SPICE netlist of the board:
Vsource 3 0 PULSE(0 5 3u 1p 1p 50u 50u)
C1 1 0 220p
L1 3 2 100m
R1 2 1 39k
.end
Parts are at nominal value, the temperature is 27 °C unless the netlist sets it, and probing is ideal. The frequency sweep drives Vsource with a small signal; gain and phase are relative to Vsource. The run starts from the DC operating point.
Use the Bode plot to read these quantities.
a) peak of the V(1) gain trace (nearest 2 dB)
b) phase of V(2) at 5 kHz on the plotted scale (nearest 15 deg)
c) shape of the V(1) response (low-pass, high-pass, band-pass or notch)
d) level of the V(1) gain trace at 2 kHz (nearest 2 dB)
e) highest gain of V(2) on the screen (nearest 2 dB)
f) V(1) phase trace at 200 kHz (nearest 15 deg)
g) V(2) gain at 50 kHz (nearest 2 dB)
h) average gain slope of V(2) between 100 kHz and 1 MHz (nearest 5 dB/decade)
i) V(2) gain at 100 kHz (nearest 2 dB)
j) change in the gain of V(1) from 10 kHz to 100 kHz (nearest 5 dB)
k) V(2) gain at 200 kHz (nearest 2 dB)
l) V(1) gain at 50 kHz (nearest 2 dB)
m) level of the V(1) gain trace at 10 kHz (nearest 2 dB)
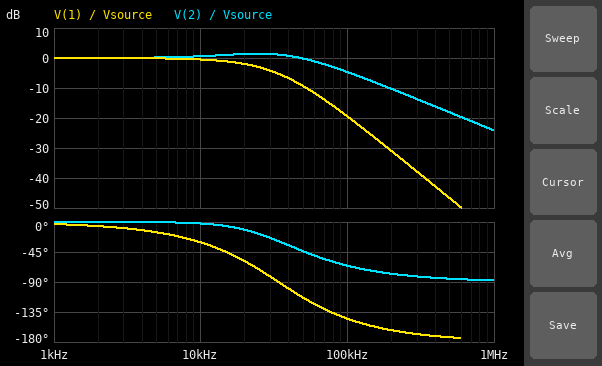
0 dB
0 deg
low-pass
0 dB
2 dB
-165 deg
0 dB
-20 dB/decade
-4 dB
-20 dB
-10 dB
-10 dB
0 dB
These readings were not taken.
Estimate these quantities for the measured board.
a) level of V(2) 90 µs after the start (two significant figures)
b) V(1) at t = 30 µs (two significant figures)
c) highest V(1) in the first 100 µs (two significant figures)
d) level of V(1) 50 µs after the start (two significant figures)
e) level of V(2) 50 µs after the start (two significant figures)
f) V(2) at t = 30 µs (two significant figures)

5.0 V
5.0 V
5.0 V
5.0 V
5.0 V
5.1 V
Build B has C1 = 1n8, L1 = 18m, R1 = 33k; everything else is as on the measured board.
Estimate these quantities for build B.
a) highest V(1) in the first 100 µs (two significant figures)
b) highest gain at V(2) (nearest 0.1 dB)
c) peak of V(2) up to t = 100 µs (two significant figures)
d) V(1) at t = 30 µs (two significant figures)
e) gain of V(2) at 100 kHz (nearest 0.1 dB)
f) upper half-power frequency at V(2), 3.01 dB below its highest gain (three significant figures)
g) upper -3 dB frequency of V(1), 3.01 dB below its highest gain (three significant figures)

4.0 V
0.1 dB
5.0 V
1.8 V
-0.4 dB
290 kHz
2.70 kHz
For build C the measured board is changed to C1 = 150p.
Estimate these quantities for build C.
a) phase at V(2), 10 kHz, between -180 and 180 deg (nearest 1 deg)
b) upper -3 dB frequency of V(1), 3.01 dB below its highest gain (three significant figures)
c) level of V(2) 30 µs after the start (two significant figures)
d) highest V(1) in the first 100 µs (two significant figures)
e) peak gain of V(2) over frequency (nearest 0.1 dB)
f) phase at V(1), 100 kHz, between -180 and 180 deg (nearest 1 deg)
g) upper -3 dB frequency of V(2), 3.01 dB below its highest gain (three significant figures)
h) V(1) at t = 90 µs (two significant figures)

-1 deg
38.3 kHz
5.0 V
5.1 V
1.9 dB
-143 deg
68.4 kHz
5.0 V
